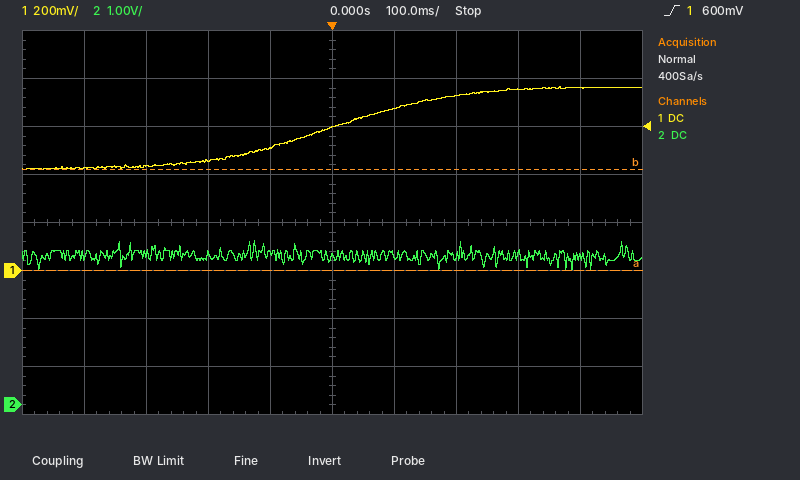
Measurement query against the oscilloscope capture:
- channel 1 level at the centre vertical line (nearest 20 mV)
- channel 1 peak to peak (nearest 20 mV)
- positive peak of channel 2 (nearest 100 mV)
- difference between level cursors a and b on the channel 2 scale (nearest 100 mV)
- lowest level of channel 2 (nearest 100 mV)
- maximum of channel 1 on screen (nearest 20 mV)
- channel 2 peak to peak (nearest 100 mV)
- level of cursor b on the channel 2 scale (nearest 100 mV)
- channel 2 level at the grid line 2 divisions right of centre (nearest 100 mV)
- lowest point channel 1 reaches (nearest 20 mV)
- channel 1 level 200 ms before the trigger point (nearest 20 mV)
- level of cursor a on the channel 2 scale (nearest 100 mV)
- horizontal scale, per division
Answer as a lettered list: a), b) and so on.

a) 600 mV
b) 340 mV
c) 3.4 V
d) 2.1 V
e) 2.8 V
f) 760 mV
g) 600 mV
h) 4.9 V
i) 3.1 V
j) 420 mV
k) 460 mV
l) 2.8 V
m) 100 ms
